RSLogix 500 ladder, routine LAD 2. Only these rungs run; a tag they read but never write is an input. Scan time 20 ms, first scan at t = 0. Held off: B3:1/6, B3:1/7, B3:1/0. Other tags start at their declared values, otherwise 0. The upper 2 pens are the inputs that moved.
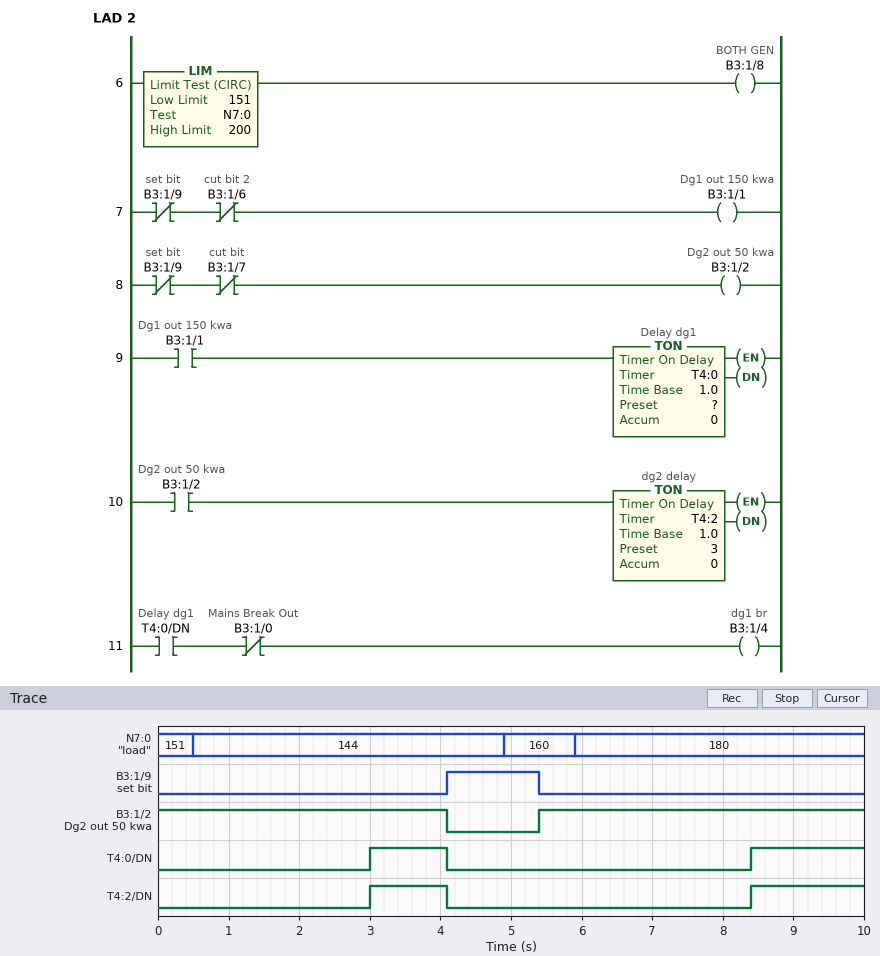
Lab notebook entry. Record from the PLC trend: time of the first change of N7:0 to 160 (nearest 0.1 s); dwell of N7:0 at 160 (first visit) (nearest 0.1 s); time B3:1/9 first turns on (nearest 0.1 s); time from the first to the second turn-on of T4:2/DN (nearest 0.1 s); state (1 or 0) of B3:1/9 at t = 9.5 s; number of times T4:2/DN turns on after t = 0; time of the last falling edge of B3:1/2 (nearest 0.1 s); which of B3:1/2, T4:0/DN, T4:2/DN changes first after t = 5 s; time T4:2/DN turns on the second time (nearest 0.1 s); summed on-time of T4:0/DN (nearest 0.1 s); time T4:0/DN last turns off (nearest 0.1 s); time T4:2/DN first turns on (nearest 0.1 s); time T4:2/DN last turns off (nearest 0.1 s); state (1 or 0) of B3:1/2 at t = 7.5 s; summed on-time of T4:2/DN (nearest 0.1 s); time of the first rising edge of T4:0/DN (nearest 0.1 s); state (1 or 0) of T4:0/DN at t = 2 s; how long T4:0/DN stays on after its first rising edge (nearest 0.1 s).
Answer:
4.9 s
1.0 s
4.1 s
5.4 s
0
2
4.1 s
B3:1/2
8.4 s
2.7 s
4.1 s
3.0 s
4.1 s
1
2.7 s
3.0 s
0
1.1 s
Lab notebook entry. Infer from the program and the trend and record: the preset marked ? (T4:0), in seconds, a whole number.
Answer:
3 s
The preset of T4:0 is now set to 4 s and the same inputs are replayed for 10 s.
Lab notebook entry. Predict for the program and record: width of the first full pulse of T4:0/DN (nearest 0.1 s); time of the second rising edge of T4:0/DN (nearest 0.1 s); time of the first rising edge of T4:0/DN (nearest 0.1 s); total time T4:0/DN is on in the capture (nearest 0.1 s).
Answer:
0.1 s
9.4 s
4.0 s
0.7 s
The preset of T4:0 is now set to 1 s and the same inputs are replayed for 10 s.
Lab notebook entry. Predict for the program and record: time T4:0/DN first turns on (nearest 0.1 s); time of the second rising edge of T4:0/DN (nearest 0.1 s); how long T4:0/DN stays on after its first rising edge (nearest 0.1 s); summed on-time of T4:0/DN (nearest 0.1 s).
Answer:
1.0 s
6.4 s
3.1 s
6.7 s
